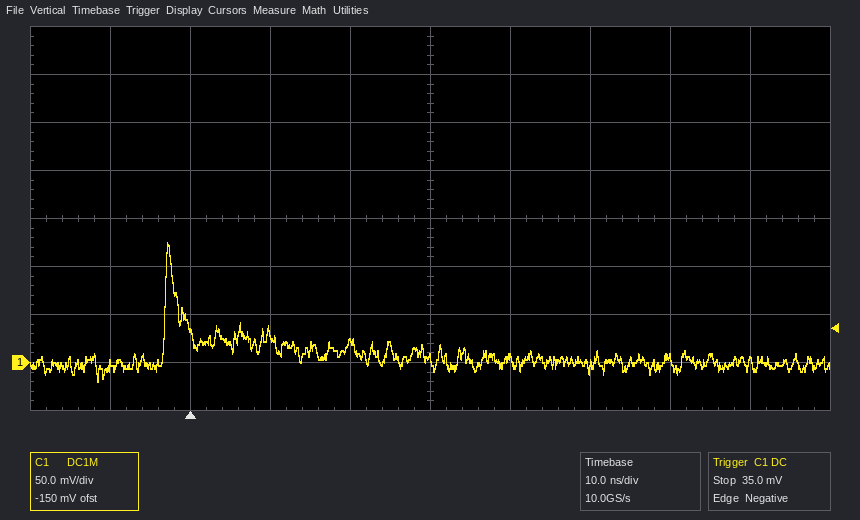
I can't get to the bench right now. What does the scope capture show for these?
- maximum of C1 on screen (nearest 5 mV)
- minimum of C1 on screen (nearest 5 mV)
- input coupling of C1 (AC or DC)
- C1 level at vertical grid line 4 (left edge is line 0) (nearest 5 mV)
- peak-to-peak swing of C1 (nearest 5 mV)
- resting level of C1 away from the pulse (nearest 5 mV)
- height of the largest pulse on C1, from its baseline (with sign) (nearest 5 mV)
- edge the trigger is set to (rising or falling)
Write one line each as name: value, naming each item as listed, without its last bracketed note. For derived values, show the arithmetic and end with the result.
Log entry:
maximum of C1 on screen: 125 mV
minimum of C1 on screen: -20 mV
input coupling of C1: DC
C1 level at vertical grid line 4 (left edge is line 0): 20 mV
peak-to-peak swing of C1: 125 mV − (-20 mV) = 145 mV
resting level of C1 away from the pulse: 0 mV
height of the largest pulse on C1, from its baseline (with sign): 125 mV − (0 mV) = +125 mV
edge the trigger is set to: falling
